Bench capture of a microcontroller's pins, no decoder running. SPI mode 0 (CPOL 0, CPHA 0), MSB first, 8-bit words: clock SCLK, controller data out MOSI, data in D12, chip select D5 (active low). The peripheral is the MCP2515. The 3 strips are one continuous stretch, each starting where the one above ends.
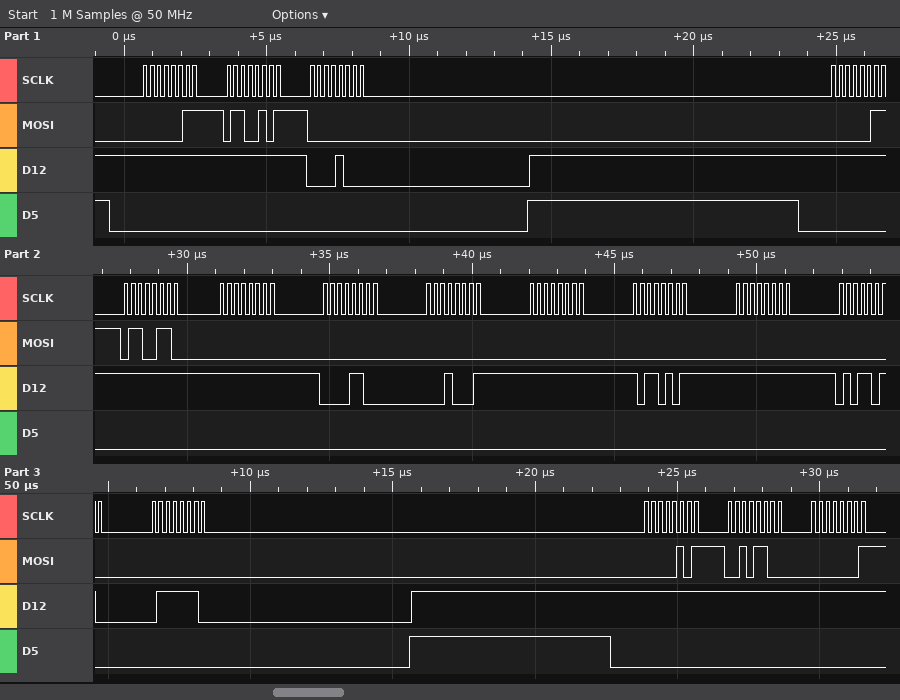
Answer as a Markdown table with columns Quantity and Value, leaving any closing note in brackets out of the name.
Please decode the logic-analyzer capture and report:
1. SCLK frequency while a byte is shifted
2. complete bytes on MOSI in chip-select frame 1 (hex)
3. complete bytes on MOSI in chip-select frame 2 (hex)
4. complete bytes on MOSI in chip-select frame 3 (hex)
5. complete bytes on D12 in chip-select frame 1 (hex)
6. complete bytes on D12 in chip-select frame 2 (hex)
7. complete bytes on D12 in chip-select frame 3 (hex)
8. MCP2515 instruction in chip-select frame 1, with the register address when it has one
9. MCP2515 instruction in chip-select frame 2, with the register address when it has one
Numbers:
| Quantity | Value |
|---|---|
| SCLK frequency while a byte is shifted | 4 MHz |
| complete bytes on MOSI in chip-select frame 1 | 03 65 00 |
| complete bytes on MOSI in chip-select frame 2 | 03 66 00 00 00 00 00 00 00 00 |
| complete bytes on MOSI in chip-select frame 3 | 05 2C 01 |
| complete bytes on D12 in chip-select frame 1 | FF FF 08 |
| complete bytes on D12 in chip-select frame 2 | FF FF FF 0C 11 FF B5 FF 5A 7E |
| complete bytes on D12 in chip-select frame 3 | FF FF FF |
| MCP2515 instruction in chip-select frame 1, with the register address when it has one | READ 0x65 |
| MCP2515 instruction in chip-select frame 2, with the register address when it has one | READ 0x66 |
